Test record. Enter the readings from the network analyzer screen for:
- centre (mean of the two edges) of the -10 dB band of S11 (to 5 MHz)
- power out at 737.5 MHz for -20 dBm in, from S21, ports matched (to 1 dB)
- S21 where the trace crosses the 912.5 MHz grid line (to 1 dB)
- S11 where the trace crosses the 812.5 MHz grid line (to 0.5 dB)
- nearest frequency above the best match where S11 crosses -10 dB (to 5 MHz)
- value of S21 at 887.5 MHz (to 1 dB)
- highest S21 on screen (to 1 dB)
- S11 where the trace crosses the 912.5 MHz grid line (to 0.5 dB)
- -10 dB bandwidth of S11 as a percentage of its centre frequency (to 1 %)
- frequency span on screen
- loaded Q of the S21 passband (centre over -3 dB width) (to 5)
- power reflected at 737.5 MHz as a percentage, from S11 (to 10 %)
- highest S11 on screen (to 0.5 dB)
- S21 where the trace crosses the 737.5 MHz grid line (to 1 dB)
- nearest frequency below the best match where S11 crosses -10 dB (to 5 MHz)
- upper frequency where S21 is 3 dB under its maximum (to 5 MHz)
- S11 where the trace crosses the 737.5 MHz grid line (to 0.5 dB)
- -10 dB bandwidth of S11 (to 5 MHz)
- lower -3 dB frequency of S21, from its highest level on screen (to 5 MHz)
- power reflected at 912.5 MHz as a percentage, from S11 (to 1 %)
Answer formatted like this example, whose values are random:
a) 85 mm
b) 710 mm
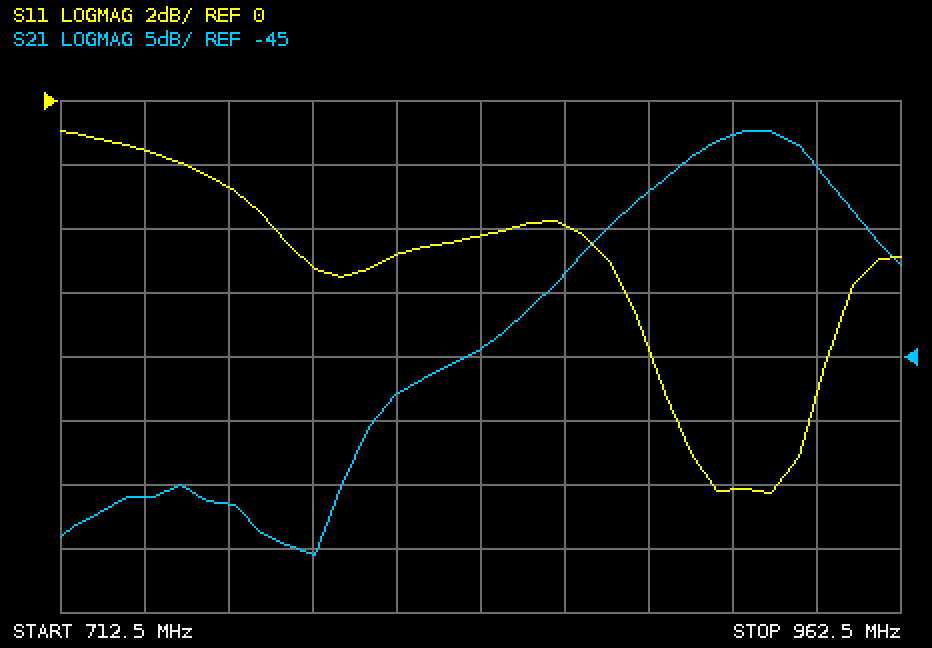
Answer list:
a) 915 MHz
b) -76 dBm
c) -28 dB
d) -5.0 dB
e) 935 MHz
f) -32 dB
g) -27 dB
h) -12.0 dB
i) 4 %
j) 250 MHz
k) 20
l) 70 %
m) -1.0 dB
n) -56 dB
o) 895 MHz
p) 940 MHz
q) -1.5 dB
r) 40 MHz
s) 895 MHz
t) 6 %
